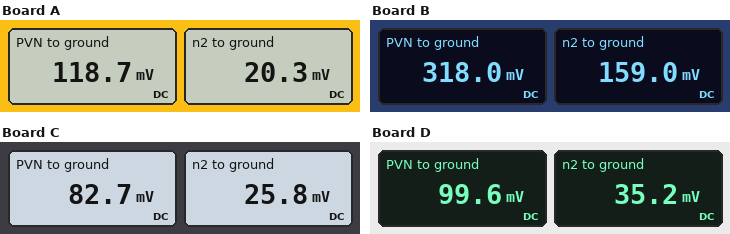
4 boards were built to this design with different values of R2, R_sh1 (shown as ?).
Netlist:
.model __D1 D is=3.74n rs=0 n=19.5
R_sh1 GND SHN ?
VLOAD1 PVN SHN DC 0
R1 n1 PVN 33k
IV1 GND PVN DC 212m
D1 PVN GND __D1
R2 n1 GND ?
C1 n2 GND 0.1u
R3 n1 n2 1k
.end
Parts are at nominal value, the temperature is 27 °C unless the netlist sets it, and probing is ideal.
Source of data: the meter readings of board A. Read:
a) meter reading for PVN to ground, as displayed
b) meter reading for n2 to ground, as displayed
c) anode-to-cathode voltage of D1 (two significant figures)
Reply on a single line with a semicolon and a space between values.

118.7 mV; 20.3 mV; 120 mV
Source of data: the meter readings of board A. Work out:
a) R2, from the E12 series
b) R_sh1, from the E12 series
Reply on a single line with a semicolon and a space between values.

6.8 kΩ; 0.56 Ω
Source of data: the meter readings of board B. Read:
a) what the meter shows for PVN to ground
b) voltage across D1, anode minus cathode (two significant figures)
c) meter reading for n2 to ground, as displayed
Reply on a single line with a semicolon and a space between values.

318.0 mV; 320 mV; 159.0 mV
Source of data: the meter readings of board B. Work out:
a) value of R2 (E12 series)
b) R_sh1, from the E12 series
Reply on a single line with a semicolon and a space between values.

33 kΩ; 1.5 Ω
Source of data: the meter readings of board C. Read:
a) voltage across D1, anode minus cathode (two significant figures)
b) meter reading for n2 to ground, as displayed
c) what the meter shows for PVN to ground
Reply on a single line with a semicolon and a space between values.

83 mV; 25.8 mV; 82.7 mV
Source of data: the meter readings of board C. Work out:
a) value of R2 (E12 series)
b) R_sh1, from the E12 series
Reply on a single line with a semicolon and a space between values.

15 kΩ; 0.39 Ω
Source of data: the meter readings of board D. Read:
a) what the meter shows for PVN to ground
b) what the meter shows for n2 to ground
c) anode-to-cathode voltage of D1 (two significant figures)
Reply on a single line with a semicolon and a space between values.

99.6 mV; 35.2 mV; 100 mV
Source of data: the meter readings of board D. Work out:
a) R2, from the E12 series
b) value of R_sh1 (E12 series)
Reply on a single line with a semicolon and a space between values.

18 kΩ; 0.47 Ω
